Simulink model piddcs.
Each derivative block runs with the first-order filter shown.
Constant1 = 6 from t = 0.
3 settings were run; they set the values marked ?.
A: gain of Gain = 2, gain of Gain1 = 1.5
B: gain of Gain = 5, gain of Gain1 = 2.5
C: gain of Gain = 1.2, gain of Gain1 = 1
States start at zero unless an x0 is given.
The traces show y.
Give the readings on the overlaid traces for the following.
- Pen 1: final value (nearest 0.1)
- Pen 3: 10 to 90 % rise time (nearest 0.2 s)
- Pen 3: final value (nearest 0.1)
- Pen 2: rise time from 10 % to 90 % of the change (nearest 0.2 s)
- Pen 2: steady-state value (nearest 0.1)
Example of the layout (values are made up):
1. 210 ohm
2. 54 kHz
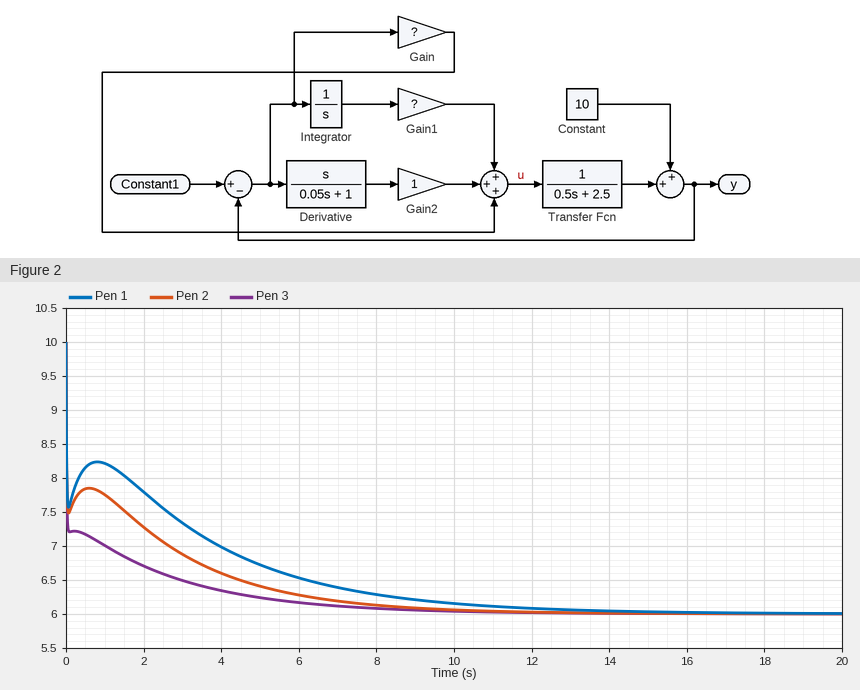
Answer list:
1. 6.0
2. 3.6 s
3. 6.0
4. 5.0 s
5. 6.0
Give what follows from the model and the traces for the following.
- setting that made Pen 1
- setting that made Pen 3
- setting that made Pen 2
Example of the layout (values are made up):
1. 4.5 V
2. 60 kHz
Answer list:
1. C
2. B
3. A
